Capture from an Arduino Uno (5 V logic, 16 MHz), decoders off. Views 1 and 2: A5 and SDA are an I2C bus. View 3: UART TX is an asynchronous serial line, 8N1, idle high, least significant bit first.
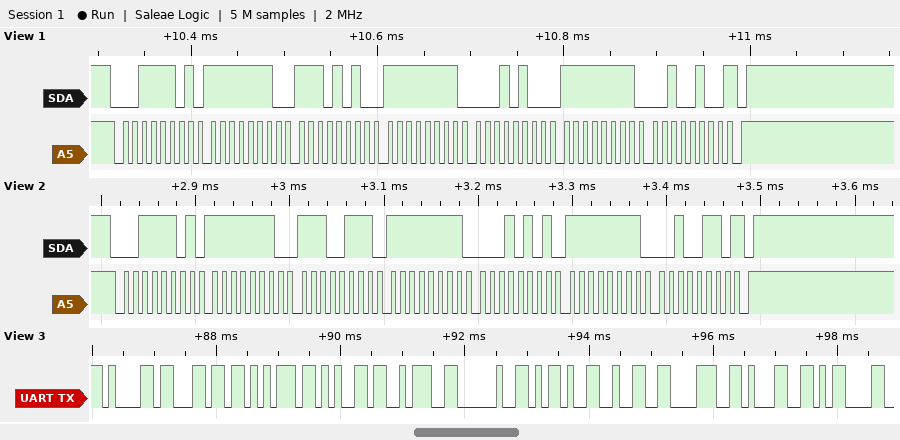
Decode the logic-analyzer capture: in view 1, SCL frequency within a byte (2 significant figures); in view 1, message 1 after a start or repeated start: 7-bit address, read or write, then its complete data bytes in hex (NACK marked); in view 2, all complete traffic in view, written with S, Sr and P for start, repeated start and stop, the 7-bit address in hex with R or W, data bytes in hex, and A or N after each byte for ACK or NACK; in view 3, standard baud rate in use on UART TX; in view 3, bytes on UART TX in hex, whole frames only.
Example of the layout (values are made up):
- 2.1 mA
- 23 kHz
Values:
- 100 kHz
- 0x1E read: FE EA FF 14 FF 24 NACK
- S 1ER A FE A E7 A FF A 15 A FF A 26 N P
- 9600 baud
- 61 6C 75 65 3A 20 2D 32 38 31 0D
